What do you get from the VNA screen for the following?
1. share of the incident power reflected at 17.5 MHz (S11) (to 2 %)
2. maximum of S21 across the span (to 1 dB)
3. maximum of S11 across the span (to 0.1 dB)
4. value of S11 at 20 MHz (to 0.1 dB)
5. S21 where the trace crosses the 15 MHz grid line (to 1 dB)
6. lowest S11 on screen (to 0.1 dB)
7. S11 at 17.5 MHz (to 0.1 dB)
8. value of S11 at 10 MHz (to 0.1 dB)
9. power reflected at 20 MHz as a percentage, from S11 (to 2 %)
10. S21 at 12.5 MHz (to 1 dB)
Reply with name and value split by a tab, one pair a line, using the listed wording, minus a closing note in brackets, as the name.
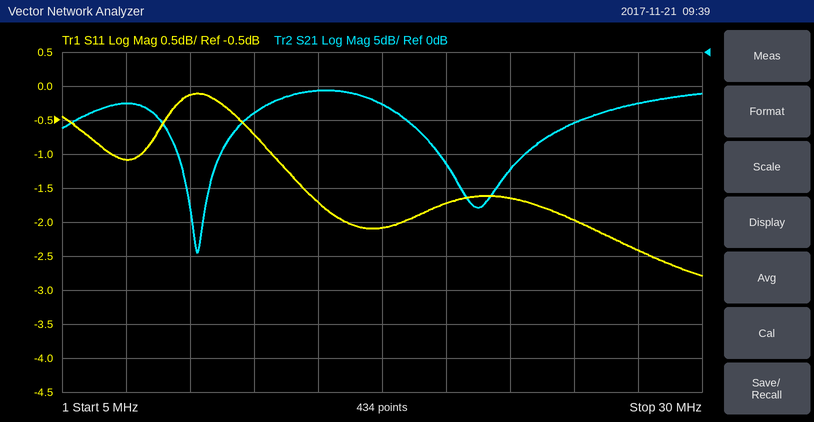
share of the incident power reflected at 17.5 MHz (S11)	62 %
maximum of S21 across the span	-6 dB
maximum of S11 across the span	-0.1 dB
value of S11 at 20 MHz	-1.7 dB
S21 where the trace crosses the 15 MHz grid line	-6 dB
lowest S11 on screen	-2.8 dB
S11 at 17.5 MHz	-2.1 dB
value of S11 at 10 MHz	-0.1 dB
power reflected at 20 MHz as a percentage, from S11	68 %
S21 at 12.5 MHz	-9 dB
